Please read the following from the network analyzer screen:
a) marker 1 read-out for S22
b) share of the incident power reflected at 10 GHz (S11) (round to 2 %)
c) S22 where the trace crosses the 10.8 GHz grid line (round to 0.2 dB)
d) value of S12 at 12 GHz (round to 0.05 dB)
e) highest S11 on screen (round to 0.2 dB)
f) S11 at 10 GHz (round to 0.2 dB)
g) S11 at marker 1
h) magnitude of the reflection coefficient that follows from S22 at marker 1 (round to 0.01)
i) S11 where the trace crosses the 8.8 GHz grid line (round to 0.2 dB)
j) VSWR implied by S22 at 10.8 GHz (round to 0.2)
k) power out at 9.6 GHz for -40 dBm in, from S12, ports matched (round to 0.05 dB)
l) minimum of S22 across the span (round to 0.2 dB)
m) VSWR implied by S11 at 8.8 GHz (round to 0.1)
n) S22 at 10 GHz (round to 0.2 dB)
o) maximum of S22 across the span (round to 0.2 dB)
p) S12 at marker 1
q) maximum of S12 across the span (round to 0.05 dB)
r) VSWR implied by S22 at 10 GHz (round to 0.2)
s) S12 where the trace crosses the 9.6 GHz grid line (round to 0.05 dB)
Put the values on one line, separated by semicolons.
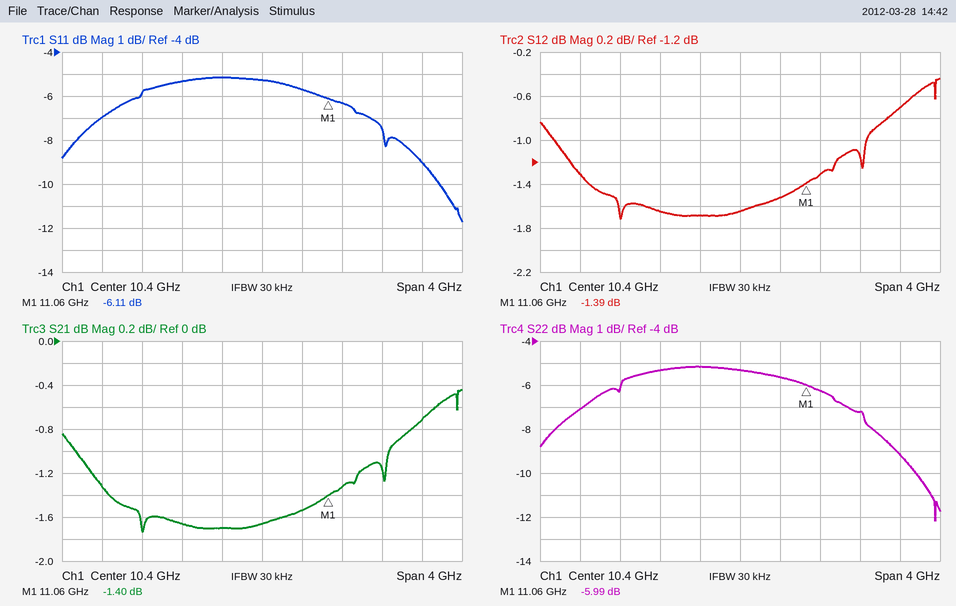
-5.99 dB; 30 %; -5.6 dB; -0.70 dB; -5.2 dB; -5.2 dB; -6.11 dB; 0.50; -7.0 dB; 3.2; -41.65 dBm; -12.2 dB; 2.6; -5.2 dB; -5.2 dB; -1.39 dB; -0.45 dB; 3.4; -1.65 dB
